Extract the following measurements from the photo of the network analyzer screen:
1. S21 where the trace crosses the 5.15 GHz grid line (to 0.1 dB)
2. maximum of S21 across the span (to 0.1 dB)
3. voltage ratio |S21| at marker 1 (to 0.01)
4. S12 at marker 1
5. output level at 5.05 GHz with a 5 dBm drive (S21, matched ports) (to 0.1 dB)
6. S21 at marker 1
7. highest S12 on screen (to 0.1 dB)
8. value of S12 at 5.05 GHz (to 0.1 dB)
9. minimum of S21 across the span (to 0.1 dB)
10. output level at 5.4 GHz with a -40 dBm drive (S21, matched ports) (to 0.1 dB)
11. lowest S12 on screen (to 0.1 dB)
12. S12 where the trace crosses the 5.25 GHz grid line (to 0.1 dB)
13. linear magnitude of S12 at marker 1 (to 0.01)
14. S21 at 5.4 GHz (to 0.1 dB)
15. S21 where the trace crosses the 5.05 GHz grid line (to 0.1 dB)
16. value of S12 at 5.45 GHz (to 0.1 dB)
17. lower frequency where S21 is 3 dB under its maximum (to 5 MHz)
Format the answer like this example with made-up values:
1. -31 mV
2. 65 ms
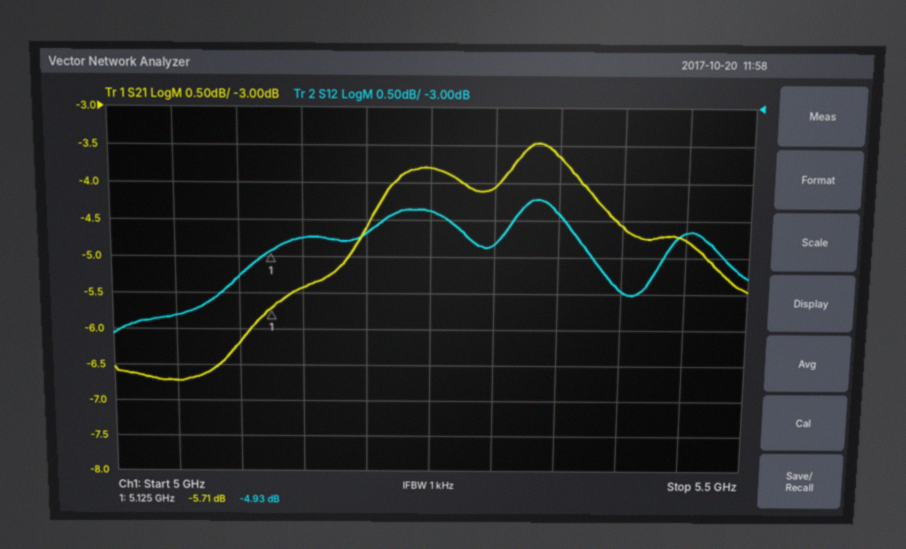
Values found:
1. -5.4 dB
2. -3.5 dB
3. 0.52
4. -4.93 dB
5. -1.7 dBm
6. -5.71 dB
7. -4.2 dB
8. -5.8 dB
9. -6.7 dB
10. -44.6 dBm
11. -6.1 dB
12. -4.4 dB
13. 0.57
14. -4.6 dB
15. -6.7 dB
16. -4.7 dB
17. 5.085 GHz
